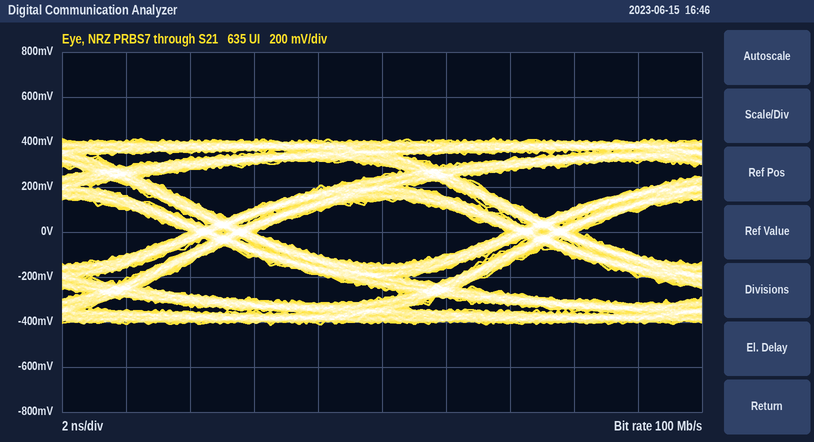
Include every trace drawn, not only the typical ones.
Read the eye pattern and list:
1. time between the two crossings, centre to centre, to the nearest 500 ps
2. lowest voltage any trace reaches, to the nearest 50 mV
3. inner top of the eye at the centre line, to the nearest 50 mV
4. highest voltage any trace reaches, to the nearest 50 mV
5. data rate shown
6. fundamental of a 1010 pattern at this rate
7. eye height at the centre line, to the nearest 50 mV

10.0 ns
-400 mV
150 mV
400 mV
100 Mb/s
50 MHz
300 mV
